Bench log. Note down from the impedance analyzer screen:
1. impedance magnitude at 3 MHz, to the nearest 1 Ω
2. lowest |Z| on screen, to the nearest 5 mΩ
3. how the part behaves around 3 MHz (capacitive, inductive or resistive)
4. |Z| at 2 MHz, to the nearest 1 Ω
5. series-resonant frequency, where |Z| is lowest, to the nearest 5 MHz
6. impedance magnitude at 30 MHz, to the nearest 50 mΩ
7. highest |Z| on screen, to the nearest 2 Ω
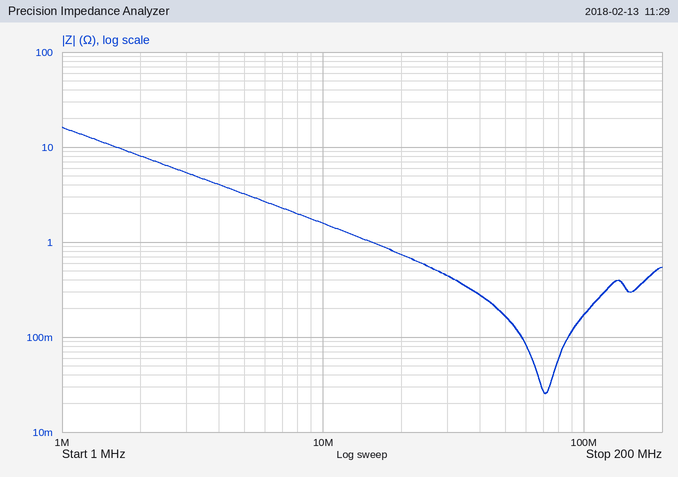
5 Ω
25 mΩ
capacitive
8 Ω
70 MHz
450 mΩ
16 Ω
